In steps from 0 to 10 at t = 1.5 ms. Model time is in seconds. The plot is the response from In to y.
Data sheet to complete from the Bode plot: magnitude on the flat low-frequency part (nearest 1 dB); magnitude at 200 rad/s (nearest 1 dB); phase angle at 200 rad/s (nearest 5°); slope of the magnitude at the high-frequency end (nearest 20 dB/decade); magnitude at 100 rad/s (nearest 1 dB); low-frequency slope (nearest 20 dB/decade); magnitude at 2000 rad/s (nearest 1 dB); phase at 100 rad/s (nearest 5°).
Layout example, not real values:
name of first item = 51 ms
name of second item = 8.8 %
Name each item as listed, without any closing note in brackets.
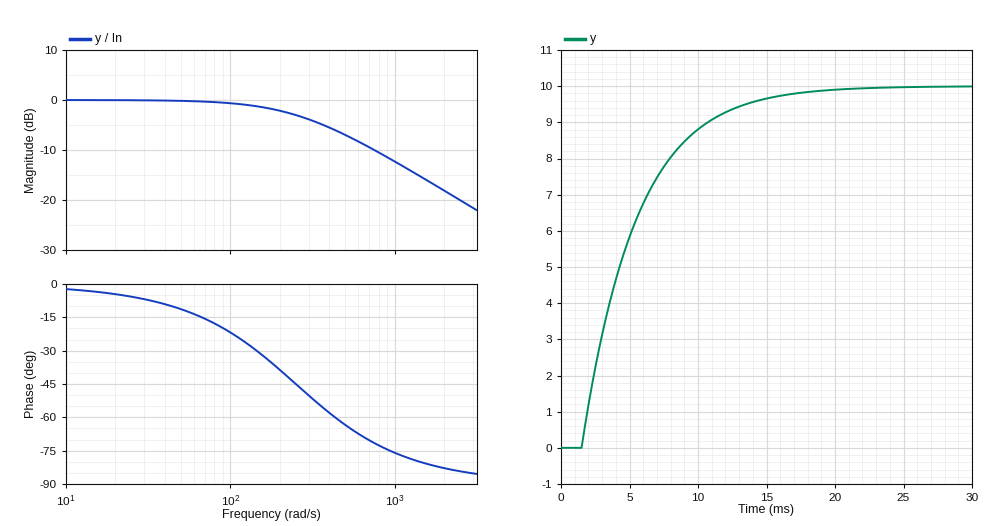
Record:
magnitude on the flat low-frequency part = 0 dB
magnitude at 200 rad/s = -2 dB
phase angle at 200 rad/s = -40°
slope of the magnitude at the high-frequency end = -20 dB/decade
magnitude at 100 rad/s = -1 dB
low-frequency slope = 0 dB/decade
magnitude at 2000 rad/s = -18 dB
phase at 100 rad/s = -20°
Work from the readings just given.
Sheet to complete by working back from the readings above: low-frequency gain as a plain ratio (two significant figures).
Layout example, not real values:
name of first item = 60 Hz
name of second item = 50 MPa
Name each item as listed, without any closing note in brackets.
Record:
low-frequency gain as a plain ratio = 1.0
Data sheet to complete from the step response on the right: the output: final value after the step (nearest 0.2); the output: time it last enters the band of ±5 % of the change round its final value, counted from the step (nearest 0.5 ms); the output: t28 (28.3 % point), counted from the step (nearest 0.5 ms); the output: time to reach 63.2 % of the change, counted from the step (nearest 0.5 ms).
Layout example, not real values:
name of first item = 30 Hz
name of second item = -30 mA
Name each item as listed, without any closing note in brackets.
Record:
the output: final value after the step = 10.0
the output: time it last enters the band of ±5 % of the change round its final value, counted from the step = 12.0 ms
the output: t28 (28.3 % point), counted from the step = 1.5 ms
the output: time to reach 63.2 % of the change, counted from the step = 4.0 ms
